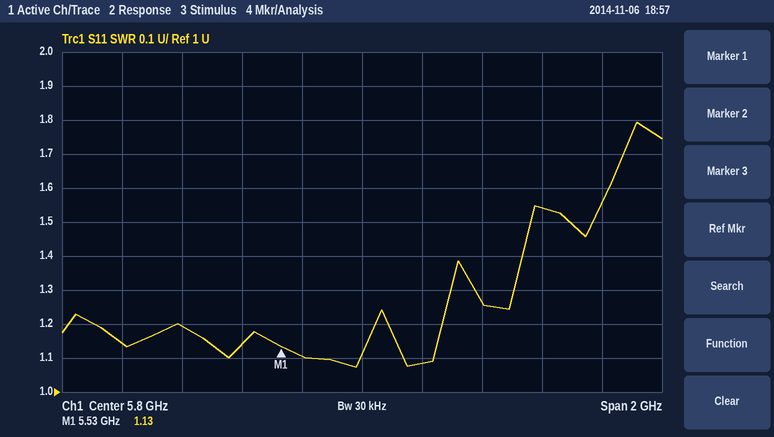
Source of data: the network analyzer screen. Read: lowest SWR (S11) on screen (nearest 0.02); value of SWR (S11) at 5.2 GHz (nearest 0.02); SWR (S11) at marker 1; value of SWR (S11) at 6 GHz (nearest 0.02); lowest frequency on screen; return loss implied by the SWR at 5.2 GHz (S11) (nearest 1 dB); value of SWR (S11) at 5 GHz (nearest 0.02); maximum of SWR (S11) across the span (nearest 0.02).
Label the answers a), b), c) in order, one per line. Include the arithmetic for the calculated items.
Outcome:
a) 1.08
b) 1.20
c) 1.13
d) 1.08
e) 4.8 GHz
f) −20 log10((1.2 − 1)/(1.2 + 1)) ≈ 21 dB
g) 1.14
h) 1.80
